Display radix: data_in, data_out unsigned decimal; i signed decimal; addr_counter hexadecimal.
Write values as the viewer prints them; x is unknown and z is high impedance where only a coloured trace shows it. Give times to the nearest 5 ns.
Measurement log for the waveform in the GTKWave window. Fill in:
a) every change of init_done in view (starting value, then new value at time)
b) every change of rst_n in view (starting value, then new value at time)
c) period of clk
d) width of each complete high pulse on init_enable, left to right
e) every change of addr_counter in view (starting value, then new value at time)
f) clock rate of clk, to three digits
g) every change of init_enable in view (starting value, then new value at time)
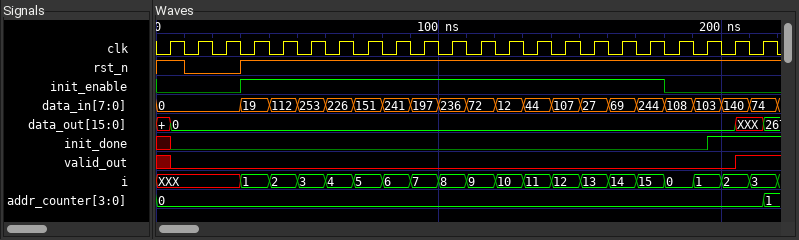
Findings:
x, 0 at 5 ns, 1 at 195 ns
1, 0 at 10 ns, 1 at 30 ns
10 ns
150 ns
0, 1 at 215 ns
100 MHz
0, 1 at 30 ns, 0 at 180 ns
